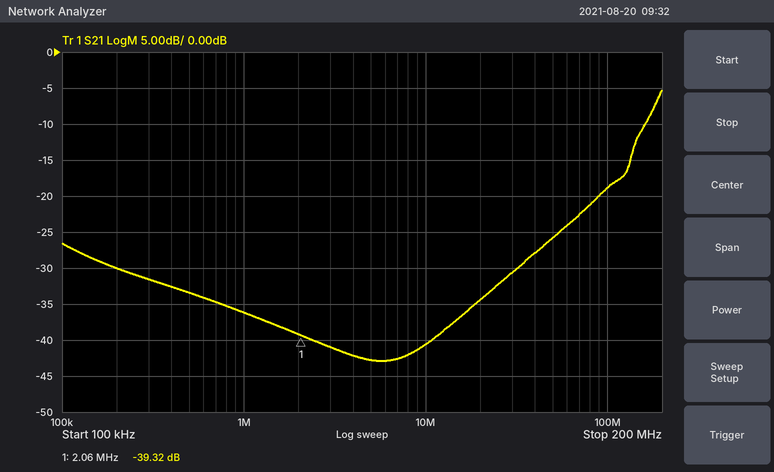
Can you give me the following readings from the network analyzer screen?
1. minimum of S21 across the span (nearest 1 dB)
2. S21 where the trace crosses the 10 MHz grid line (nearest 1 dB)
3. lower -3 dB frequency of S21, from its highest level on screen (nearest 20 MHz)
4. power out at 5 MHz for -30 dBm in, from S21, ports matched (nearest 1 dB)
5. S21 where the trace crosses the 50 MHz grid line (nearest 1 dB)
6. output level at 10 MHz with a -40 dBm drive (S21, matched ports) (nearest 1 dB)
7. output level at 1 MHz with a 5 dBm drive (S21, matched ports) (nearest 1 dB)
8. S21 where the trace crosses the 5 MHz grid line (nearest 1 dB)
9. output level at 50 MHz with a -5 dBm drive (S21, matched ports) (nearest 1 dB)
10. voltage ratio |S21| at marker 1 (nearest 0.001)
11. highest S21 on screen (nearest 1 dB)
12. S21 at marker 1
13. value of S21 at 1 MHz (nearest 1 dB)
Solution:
-43 dB
-41 dB
180 MHz
-73 dBm
-26 dB
-81 dBm
-31 dBm
-43 dB
-31 dBm
0.011
-5 dB
-39.32 dB
-36 dB
